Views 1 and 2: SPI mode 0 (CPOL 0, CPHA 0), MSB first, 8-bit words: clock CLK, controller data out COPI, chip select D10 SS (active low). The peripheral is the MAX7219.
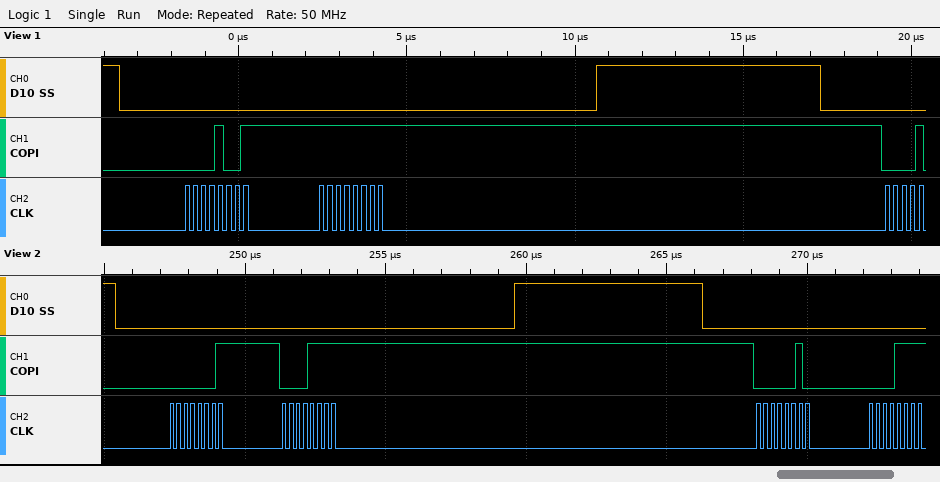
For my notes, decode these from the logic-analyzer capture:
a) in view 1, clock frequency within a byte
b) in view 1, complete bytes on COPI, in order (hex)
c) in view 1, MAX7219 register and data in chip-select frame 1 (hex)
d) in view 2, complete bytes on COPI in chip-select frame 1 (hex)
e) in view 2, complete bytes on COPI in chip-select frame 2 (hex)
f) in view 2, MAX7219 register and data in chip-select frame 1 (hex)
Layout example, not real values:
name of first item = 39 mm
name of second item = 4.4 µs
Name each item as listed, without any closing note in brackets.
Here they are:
in view 1, clock frequency within a byte = 4 MHz
in view 1, complete bytes on COPI, in order = 09 FF
in view 1, MAX7219 register and data in chip-select frame 1 = register 0x9, data 0xFF
in view 2, complete bytes on COPI in chip-select frame 1 = 0x01 0x0F
in view 2, complete bytes on COPI in chip-select frame 2 = 0x02 0x0F
in view 2, MAX7219 register and data in chip-select frame 1 = register 0x1, data 0x0F
